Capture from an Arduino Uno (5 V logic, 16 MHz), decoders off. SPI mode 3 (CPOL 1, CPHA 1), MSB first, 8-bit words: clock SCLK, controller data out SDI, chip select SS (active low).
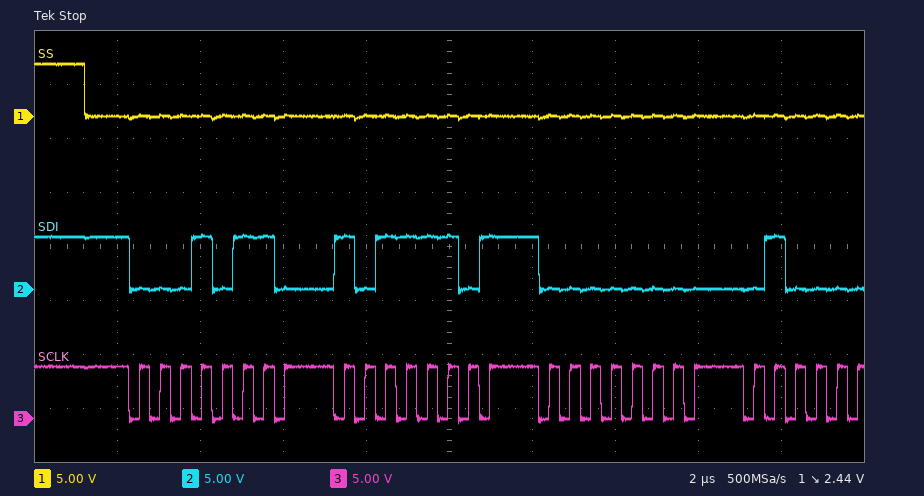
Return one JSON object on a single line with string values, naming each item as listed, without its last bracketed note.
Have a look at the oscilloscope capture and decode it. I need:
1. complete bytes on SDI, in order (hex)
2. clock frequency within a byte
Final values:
{"complete bytes on SDI, in order": "16 BD 00", "clock frequency within a byte": "2 MHz"}
